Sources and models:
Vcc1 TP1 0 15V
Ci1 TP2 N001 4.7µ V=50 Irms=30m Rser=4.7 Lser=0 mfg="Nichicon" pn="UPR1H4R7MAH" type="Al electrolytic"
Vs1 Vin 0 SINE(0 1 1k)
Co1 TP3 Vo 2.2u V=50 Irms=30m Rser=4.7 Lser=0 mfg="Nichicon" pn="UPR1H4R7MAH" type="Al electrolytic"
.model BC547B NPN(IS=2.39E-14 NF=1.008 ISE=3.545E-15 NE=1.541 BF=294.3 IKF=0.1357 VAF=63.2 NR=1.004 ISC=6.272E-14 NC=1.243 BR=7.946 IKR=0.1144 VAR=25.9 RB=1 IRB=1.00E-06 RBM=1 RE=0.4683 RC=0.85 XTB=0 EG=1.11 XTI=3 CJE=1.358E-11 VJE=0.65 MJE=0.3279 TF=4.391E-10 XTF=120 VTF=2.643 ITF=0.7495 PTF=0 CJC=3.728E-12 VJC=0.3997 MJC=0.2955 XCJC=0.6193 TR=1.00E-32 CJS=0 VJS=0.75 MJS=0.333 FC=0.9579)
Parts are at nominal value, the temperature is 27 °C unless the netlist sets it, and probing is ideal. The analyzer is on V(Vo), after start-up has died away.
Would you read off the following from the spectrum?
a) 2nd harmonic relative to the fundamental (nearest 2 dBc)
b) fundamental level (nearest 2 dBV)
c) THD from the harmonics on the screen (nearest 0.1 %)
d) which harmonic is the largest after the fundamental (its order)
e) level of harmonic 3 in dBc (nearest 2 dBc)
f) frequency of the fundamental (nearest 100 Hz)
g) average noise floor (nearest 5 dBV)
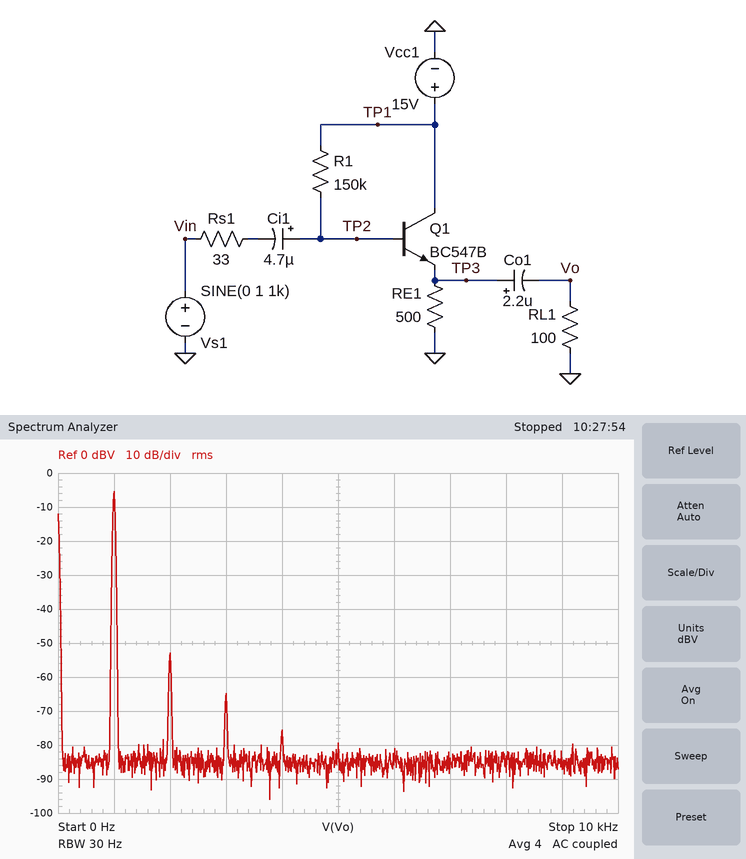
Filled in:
-48 dBc
-6 dBV
0.4 %
2
-60 dBc
1.0 kHz
-85 dBV
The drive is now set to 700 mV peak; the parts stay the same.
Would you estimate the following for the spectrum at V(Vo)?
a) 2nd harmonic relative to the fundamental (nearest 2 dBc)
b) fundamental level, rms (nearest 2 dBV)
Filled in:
-52 dBc
-8 dBV
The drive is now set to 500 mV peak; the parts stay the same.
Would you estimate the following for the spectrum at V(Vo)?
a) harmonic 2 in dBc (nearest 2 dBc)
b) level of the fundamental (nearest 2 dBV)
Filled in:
-56 dBc
-12 dBV
